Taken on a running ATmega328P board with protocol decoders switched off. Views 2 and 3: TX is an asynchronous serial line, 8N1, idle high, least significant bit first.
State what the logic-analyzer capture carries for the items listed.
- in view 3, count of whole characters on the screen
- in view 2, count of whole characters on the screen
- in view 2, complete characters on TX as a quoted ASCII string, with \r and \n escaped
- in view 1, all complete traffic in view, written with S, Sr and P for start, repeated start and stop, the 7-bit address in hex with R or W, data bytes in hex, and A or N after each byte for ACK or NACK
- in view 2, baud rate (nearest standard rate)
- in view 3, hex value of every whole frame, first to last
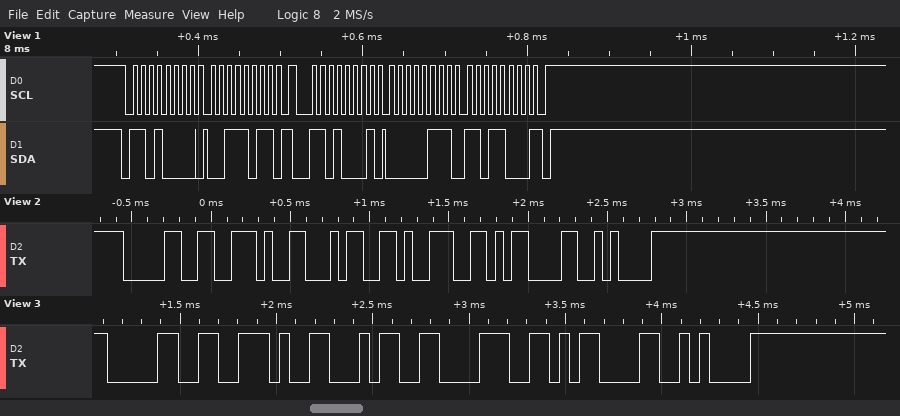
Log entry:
6
6
"0.49\r\n"
S 68W A 3B A Sr 68R A 07 A D8 N P
19200 baud
0x30 0x2E 0x34 0x38 0x0D 0x0A
